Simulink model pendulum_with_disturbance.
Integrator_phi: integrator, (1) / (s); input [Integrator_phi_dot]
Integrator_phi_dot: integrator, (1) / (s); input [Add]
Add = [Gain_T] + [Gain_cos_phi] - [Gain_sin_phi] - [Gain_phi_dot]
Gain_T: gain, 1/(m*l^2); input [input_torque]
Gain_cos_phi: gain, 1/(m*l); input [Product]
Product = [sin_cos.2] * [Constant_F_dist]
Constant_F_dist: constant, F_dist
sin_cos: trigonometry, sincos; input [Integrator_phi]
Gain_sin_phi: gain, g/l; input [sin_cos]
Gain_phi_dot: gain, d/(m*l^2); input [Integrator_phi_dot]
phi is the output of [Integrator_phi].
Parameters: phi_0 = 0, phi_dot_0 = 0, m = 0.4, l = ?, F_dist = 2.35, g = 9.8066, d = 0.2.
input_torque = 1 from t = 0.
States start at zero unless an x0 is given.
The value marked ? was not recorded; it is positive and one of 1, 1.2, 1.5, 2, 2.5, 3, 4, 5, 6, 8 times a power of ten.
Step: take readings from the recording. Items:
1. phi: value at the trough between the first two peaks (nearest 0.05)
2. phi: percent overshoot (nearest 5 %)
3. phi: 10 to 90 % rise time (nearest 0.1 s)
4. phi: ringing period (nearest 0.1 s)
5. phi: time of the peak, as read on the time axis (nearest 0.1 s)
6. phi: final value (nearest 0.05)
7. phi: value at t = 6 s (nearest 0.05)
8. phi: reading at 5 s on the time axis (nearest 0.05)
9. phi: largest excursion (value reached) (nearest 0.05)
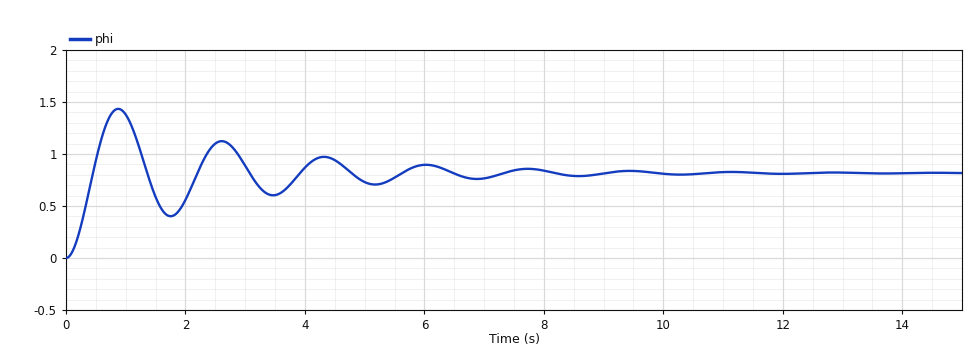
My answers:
0.40
75 %
0.3 s
1.7 s
0.9 s
0.80
0.90
0.75
1.45
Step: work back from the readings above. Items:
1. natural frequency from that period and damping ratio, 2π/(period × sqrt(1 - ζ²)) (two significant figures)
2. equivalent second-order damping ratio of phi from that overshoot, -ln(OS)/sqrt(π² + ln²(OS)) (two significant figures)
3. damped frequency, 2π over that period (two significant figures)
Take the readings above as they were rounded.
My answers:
3.7 rad/s
0.091
3.7 rad/s
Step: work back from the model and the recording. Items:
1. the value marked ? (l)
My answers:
0.8
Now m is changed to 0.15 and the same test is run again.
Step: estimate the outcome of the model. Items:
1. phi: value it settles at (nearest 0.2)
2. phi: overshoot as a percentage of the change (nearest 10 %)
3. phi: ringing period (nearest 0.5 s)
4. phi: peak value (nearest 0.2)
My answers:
1.4
50 %
1.5 s
2.2
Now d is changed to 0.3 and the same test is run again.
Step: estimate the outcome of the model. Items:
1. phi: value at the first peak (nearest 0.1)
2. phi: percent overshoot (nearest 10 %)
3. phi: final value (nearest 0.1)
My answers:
1.3
60 %
0.8
